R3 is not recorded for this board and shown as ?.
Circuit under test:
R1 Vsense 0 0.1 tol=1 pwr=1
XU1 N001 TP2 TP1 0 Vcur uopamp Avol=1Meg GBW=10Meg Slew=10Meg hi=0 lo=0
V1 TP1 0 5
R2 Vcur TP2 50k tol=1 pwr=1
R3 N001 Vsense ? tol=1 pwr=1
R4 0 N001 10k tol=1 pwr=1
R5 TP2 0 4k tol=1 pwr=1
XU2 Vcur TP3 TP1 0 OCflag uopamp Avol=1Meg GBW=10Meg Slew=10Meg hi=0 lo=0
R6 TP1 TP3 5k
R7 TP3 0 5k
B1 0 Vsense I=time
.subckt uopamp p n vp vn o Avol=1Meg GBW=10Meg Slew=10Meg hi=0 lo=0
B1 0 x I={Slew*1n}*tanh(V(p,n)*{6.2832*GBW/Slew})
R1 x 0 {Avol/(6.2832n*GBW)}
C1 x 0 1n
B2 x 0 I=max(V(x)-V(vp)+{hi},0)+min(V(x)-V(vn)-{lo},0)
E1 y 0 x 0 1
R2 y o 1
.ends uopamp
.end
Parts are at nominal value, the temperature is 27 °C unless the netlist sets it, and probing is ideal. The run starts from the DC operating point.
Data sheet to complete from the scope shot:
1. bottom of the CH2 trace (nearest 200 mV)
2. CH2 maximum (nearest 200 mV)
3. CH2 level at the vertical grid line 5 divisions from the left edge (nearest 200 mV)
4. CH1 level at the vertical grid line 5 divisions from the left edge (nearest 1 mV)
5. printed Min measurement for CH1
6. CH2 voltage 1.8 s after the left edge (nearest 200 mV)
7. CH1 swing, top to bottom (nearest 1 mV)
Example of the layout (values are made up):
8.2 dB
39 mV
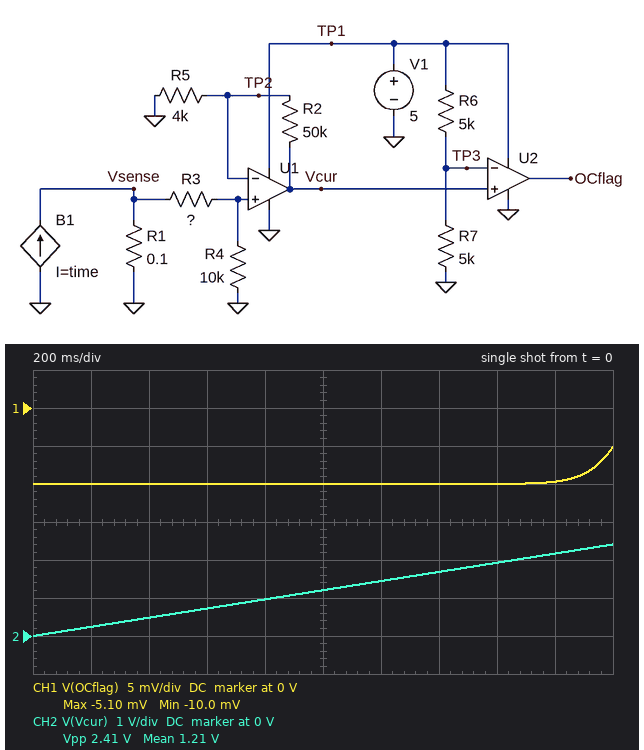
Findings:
0 V
2.4 V
1.2 V
-10 mV
-10.0 mV
2.2 V
5 mV
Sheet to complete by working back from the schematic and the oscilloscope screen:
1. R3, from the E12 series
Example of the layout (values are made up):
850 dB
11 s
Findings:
1.2 kΩ
